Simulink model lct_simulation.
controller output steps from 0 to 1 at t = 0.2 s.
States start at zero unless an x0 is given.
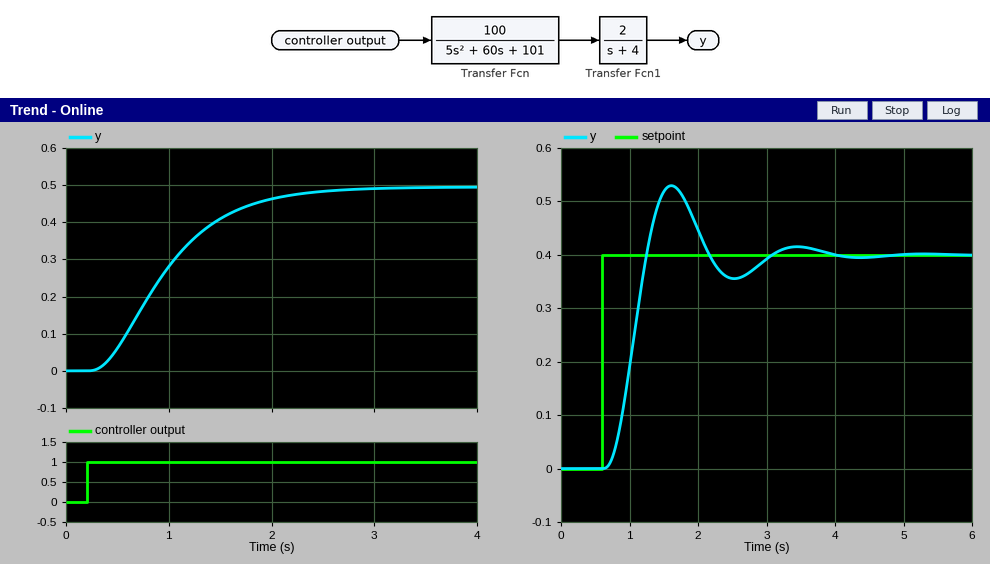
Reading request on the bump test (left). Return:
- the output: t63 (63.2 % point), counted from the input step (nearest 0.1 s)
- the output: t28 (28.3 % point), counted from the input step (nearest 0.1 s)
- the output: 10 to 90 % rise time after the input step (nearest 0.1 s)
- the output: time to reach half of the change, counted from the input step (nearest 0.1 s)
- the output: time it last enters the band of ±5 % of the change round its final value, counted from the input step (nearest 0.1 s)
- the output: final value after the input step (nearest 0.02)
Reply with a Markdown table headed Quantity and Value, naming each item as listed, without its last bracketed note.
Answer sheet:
| Quantity | Value |
|---|---|
| the output: t63 (63.2 % point), counted from the input step | 0.9 s |
| the output: t28 (28.3 % point), counted from the input step | 0.5 s |
| the output: 10 to 90 % rise time after the input step | 1.3 s |
| the output: time to reach half of the change, counted from the input step | 0.7 s |
| the output: time it last enters the band of ±5 % of the change round its final value, counted from the input step | 1.9 s |
| the output: final value after the input step | 0.50 |
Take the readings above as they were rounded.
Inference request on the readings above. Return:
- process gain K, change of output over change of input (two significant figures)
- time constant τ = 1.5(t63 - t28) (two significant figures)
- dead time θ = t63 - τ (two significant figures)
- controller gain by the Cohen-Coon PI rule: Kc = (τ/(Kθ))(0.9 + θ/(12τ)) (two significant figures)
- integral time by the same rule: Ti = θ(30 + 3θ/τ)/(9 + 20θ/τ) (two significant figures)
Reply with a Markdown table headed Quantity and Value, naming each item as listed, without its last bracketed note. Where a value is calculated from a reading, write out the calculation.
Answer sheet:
| Quantity | Value |
|---|---|
| process gain K, change of output over change of input | (0.5 - 0) / 1 = 0.50 |
| time constant τ = 1.5(t63 - t28) | 1.5 × (0.9 - 0.5) = 0.60 s |
| dead time θ = t63 - τ | 0.9 - 0.6 = 0.30 s |
| controller gain by the Cohen-Coon PI rule: Kc = (τ/(Kθ))(0.9 + θ/(12τ)) | 0.6 / (0.5 × 0.3) × (0.9 + 0.3 / (12 × 0.6)) = 3.8 |
| integral time by the same rule: Ti = θ(30 + 3θ/τ)/(9 + 20θ/τ) | 0.3 × (30 + 3 × 0.3 / 0.6) / (9 + 20 × 0.3 / 0.6) = 0.50 s |
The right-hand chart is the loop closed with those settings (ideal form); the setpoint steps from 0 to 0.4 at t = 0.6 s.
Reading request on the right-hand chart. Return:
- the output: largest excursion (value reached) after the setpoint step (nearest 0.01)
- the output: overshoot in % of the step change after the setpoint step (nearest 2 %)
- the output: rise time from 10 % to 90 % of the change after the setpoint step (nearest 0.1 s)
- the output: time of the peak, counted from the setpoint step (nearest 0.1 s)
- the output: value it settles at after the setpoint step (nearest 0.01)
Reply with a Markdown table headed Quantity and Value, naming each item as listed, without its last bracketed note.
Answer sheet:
| Quantity | Value |
|---|---|
| the output: largest excursion (value reached) after the setpoint step | 0.53 |
| the output: overshoot in % of the step change after the setpoint step | 32 % |
| the output: rise time from 10 % to 90 % of the change after the setpoint step | 0.4 s |
| the output: time of the peak, counted from the setpoint step | 1.0 s |
| the output: value it settles at after the setpoint step | 0.40 |
